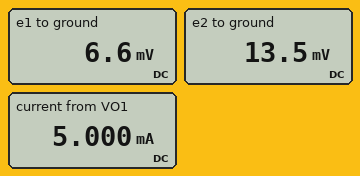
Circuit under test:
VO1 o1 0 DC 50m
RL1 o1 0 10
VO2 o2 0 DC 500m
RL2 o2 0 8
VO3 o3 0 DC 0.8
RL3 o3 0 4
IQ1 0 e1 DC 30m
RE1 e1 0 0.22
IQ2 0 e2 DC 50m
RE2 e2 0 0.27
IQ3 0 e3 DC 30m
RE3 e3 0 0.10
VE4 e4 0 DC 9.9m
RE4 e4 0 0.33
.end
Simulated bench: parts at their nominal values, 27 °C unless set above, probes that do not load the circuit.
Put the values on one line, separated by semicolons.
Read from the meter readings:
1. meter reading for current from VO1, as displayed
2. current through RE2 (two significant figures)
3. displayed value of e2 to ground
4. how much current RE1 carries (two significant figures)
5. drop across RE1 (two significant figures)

5.000 mA; 50 mA; 13.5 mV; 30 mA; 6.6 mV
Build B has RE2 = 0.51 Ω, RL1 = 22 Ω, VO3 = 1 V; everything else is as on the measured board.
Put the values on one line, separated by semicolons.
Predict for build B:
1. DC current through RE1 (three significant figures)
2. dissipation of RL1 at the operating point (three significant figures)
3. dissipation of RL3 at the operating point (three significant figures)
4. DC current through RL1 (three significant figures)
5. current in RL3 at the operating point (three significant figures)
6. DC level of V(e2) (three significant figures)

30.0 mA; 114 µW; 250 mW; 2.27 mA; 250 mA; 25.5 mV
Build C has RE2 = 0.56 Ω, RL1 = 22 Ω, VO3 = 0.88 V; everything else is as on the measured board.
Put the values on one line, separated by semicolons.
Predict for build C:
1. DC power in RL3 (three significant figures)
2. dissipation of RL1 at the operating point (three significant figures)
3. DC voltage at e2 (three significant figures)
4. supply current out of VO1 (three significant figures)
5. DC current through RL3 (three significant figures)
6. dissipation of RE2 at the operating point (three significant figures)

194 mW; 114 µW; 28.0 mV; 2.27 mA; 220 mA; 1.40 mW
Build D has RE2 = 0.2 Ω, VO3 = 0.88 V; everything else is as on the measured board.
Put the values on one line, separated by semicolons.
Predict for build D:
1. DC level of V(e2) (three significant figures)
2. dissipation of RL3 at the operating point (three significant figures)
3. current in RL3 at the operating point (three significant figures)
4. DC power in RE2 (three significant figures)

10.0 mV; 194 mW; 220 mA; 500 µW
